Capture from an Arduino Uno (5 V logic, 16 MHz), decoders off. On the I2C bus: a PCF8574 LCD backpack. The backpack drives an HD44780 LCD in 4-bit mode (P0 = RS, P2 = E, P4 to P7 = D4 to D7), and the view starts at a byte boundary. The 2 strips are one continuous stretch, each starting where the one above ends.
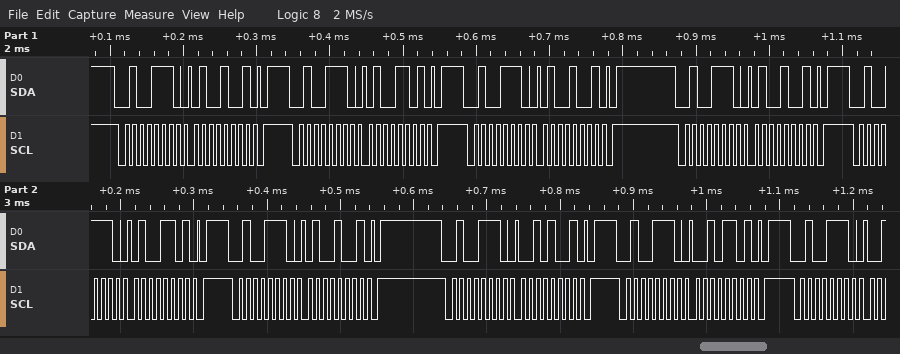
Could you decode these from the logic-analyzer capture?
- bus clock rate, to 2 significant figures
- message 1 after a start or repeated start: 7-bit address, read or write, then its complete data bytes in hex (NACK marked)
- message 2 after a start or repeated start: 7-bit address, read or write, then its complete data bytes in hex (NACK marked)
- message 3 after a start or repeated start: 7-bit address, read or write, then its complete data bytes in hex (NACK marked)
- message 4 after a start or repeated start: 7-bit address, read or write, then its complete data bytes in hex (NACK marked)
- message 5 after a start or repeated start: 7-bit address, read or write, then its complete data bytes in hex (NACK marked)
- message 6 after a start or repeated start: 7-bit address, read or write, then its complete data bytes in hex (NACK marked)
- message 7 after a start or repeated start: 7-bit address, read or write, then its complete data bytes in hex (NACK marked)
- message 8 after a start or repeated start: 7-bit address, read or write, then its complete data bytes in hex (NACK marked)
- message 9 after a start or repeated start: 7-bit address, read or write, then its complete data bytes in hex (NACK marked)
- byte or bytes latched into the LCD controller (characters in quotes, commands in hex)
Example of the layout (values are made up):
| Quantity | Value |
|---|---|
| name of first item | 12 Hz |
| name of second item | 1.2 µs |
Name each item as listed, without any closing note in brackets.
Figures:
| Quantity | Value |
|---|---|
| bus clock rate, to 2 significant figures | 100 kHz |
| message 1 after a start or repeated start: 7-bit address, read or write, then its complete data bytes in hex | 0x27 write: 49 |
| message 2 after a start or repeated start: 7-bit address, read or write, then its complete data bytes in hex | 0x27 write: 4D |
| message 3 after a start or repeated start: 7-bit address, read or write, then its complete data bytes in hex | 0x27 write: 49 |
| message 4 after a start or repeated start: 7-bit address, read or write, then its complete data bytes in hex | 0x27 write: 49 |
| message 5 after a start or repeated start: 7-bit address, read or write, then its complete data bytes in hex | 0x27 write: 4D |
| message 6 after a start or repeated start: 7-bit address, read or write, then its complete data bytes in hex | 0x27 write: 49 |
| message 7 after a start or repeated start: 7-bit address, read or write, then its complete data bytes in hex | 0x27 write: 29 |
| message 8 after a start or repeated start: 7-bit address, read or write, then its complete data bytes in hex | 0x27 write: 2D |
| message 9 after a start or repeated start: 7-bit address, read or write, then its complete data bytes in hex | 0x27 write |
| byte or bytes latched into the LCD controller | 'D' |
